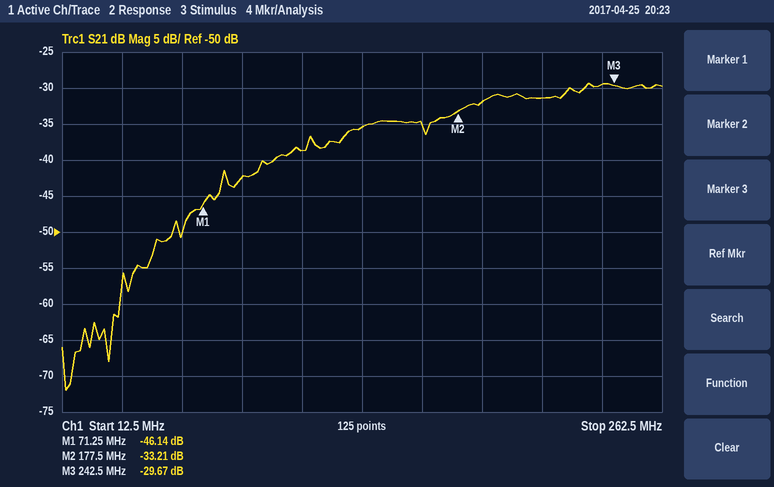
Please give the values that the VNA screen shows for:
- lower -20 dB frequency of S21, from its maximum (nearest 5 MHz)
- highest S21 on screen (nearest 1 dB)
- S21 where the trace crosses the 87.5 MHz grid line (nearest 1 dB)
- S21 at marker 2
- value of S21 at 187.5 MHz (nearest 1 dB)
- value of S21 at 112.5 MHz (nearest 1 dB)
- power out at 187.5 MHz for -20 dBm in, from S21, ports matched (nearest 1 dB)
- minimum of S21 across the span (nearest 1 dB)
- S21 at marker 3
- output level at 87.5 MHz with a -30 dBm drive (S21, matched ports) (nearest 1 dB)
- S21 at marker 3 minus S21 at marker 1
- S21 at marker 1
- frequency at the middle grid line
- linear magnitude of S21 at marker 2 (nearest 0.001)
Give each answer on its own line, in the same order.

65 MHz
-29 dB
-42 dB
-33.21 dB
-32 dB
-39 dB
-52 dBm
-72 dB
-29.67 dB
-72 dBm
16.47 dB
-46.14 dB
137.5 MHz
0.022
